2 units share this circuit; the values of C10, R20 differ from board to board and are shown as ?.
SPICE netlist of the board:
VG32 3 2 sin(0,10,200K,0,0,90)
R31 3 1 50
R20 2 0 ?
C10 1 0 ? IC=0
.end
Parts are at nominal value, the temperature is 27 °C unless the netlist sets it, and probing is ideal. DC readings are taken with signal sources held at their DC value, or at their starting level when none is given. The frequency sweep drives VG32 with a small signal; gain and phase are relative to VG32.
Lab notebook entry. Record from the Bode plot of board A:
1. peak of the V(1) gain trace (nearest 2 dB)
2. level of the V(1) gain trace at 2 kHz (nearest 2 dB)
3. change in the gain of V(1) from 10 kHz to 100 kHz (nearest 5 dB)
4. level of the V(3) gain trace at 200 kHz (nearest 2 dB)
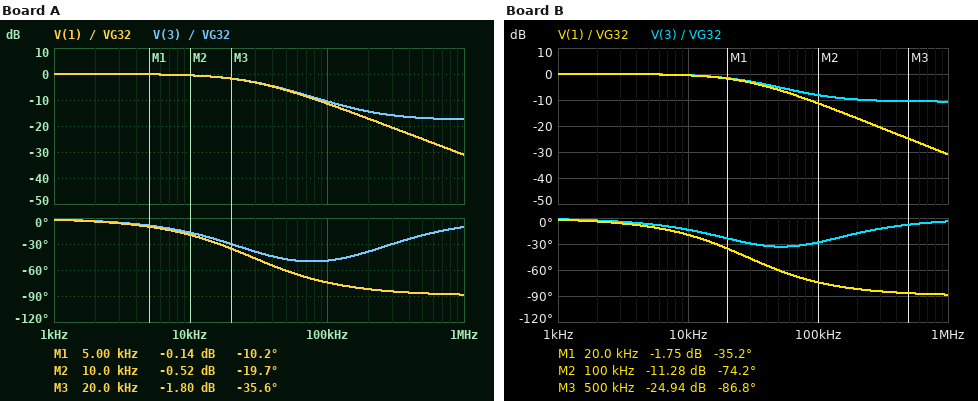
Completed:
0 dB
0 dB
-10 dB
-14 dB
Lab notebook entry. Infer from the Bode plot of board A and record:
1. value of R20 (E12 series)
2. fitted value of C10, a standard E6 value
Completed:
330 Ω
15 nF
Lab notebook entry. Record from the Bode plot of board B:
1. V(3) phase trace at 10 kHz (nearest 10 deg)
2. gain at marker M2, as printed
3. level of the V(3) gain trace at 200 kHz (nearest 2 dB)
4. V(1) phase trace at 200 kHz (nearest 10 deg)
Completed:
-10 deg
-11.28 dB
-10 dB
-80 deg
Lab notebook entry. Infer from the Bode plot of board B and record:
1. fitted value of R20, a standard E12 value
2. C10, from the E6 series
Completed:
120 Ω
33 nF
